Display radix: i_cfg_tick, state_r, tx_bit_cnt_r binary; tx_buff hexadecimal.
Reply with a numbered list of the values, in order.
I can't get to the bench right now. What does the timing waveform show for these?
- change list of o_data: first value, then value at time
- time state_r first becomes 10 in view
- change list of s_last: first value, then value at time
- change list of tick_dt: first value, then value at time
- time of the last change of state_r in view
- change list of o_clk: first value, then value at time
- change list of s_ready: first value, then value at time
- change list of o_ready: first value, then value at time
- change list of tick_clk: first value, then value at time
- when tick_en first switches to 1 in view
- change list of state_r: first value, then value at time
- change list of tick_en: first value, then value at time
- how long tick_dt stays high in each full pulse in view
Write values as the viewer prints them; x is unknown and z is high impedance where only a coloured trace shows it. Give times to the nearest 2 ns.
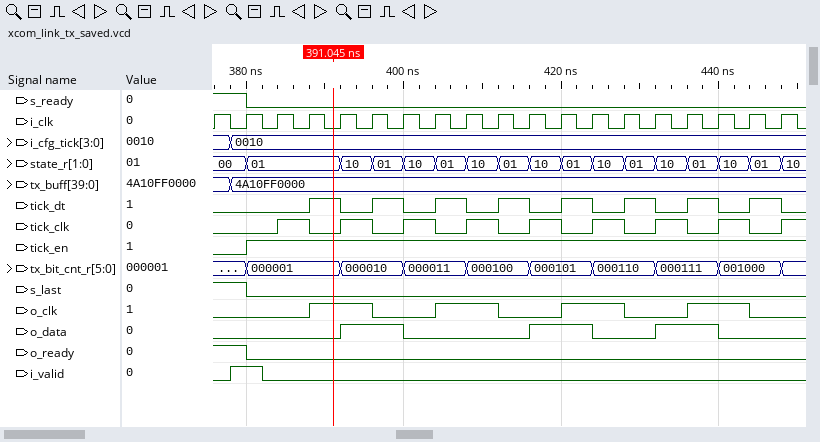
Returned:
1. 0, 1 at 392 ns, 0 at 400 ns, 1 at 416 ns, 0 at 424 ns, 1 at 432 ns, 0 at 440 ns
2. 392 ns
3. 1, 0 at 380 ns
4. 0, 1 at 388 ns, 0 at 392 ns, 1 at 396 ns, 0 at 400 ns, 1 at 404 ns, 0 at 408 ns, 1 at 412 ns, 0 at 416 ns, 1 at 420 ns, 0 at 424 ns, 1 at 428 ns, 0 at 432 ns, 1 at 436 ns, 0 at 440 ns, 1 at 444 ns, 0 at 448 ns
5. 448 ns
6. 0, 1 at 388 ns, 0 at 396 ns, 1 at 404 ns, 0 at 412 ns, 1 at 420 ns, 0 at 428 ns, 1 at 436 ns, 0 at 444 ns
7. 1, 0 at 380 ns
8. 1, 0 at 380 ns
9. 0, 1 at 384 ns, 0 at 388 ns, 1 at 392 ns, 0 at 396 ns, 1 at 400 ns, 0 at 404 ns, 1 at 408 ns, 0 at 412 ns, 1 at 416 ns, 0 at 420 ns, 1 at 424 ns, 0 at 428 ns, 1 at 432 ns, 0 at 436 ns, 1 at 440 ns, 0 at 444 ns, 1 at 448 ns
10. 380 ns
11. 00, 01 at 380 ns, 10 at 392 ns, 01 at 396 ns, 10 at 400 ns, 01 at 404 ns, 10 at 408 ns, 01 at 412 ns, 10 at 416 ns, 01 at 420 ns, 10 at 424 ns, 01 at 428 ns, 10 at 432 ns, 01 at 436 ns, 10 at 440 ns, 01 at 444 ns, 10 at 448 ns
12. 0, 1 at 380 ns
13. 4 ns, 4 ns, 4 ns, 4 ns, 4 ns, 4 ns, 4 ns, 4 ns
